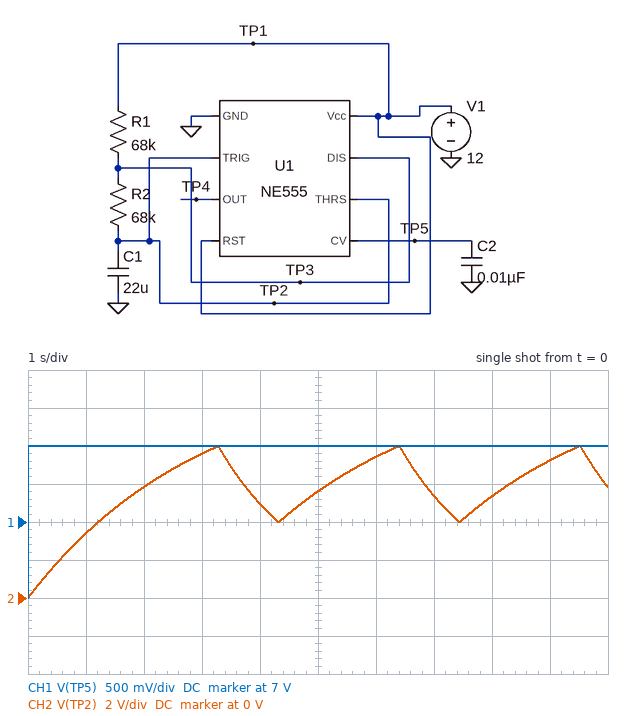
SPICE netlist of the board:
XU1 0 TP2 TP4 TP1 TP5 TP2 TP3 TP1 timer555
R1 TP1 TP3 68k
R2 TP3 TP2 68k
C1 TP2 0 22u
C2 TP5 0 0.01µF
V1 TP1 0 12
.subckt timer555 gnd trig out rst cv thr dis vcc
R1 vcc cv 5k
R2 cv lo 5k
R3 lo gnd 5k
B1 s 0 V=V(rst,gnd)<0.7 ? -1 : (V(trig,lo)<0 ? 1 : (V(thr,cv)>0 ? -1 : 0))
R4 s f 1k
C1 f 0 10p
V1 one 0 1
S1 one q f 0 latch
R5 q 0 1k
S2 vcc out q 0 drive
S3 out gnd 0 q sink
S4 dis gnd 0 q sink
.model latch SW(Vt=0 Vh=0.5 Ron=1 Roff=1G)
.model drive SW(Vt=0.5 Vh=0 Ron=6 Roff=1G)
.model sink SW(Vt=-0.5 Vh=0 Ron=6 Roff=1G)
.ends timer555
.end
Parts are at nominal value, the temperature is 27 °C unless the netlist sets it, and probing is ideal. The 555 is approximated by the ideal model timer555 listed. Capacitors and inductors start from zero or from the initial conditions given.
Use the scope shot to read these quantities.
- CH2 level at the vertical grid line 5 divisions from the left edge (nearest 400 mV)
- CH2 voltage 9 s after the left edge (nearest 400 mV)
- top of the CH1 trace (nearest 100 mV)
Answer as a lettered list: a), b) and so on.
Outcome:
a) 5.6 V
b) 7.2 V
c) 8.0 V
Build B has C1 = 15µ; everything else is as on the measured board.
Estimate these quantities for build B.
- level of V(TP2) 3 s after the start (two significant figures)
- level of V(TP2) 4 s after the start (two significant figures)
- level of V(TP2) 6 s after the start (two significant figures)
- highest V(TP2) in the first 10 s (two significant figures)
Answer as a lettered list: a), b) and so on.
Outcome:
a) 4.2 V
b) 7.2 V
c) 6.9 V
d) 8.0 V
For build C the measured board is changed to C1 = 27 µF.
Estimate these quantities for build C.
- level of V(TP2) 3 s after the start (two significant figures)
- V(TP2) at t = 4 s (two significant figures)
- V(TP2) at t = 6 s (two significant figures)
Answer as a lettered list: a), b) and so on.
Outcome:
a) 6.7 V
b) 8.0 V
c) 5.4 V
